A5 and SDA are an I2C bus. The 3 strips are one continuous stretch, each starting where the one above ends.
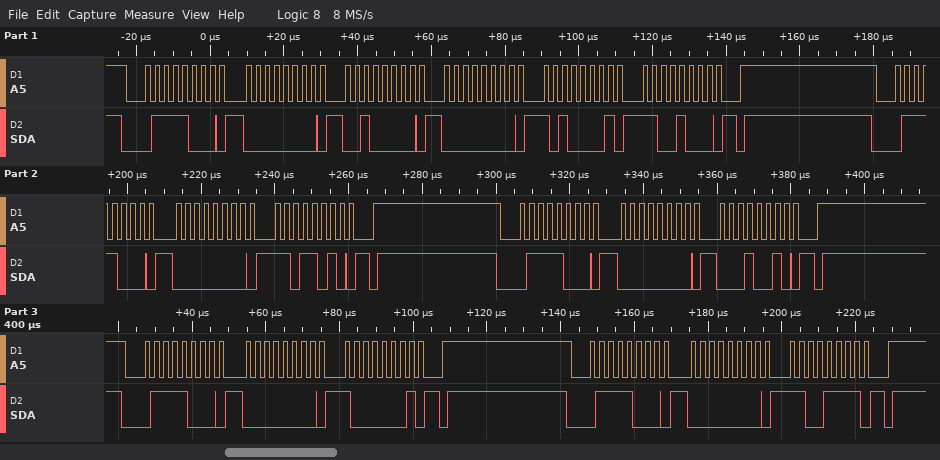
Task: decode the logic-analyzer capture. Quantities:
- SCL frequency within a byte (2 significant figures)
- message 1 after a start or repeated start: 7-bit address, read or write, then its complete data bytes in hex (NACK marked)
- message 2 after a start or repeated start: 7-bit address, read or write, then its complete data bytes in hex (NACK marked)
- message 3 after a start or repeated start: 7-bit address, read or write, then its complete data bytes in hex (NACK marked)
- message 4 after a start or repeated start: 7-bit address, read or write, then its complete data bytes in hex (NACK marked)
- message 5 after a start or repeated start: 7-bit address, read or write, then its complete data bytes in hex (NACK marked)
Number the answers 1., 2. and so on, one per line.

1. 400 kHz
2. 0x3C write: 00 20 00 A1 C8
3. 0x3C write: 00 DA
4. 0x3C write: 00 12
5. 0x3C write: 00 81
6. 0x3C write: 00 CF
